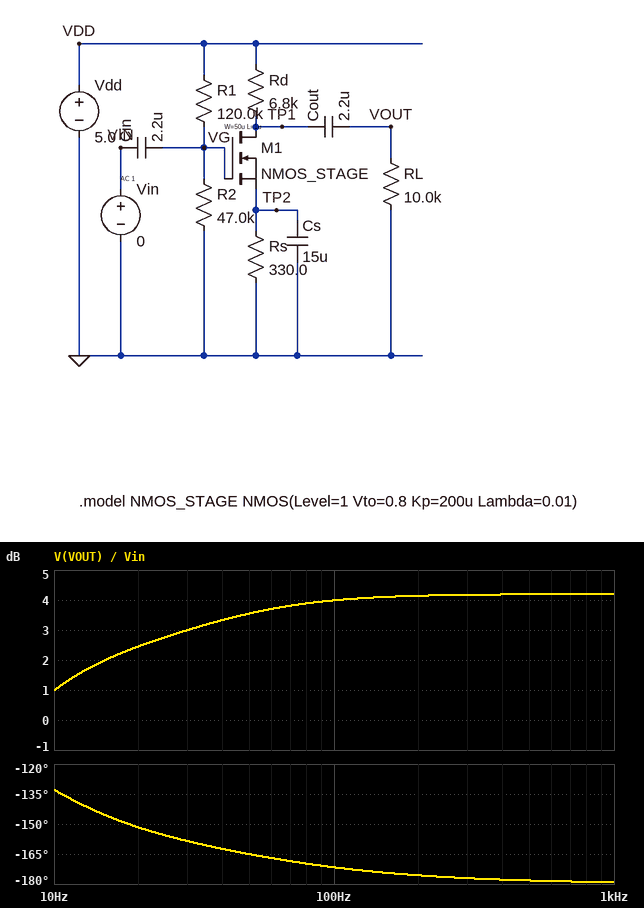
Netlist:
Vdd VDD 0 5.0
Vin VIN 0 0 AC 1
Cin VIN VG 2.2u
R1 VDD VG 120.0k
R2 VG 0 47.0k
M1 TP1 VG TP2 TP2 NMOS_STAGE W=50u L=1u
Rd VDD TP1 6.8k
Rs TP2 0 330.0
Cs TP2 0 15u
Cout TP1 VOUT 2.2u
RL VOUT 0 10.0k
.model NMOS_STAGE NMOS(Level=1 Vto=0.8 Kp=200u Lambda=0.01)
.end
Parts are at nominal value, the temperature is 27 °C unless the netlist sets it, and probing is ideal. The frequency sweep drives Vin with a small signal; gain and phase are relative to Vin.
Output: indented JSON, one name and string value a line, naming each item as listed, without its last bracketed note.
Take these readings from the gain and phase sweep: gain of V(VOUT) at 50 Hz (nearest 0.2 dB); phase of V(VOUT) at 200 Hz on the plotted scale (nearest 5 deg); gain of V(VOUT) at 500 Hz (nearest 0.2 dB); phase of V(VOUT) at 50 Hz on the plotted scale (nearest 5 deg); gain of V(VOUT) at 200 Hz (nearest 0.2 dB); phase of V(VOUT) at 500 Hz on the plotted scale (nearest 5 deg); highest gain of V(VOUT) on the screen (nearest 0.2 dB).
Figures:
{
  "gain of V(VOUT) at 50 Hz": "3.6 dB",
  "phase of V(VOUT) at 200 Hz on the plotted scale": "-175 deg",
  "gain of V(VOUT) at 500 Hz": "4.2 dB",
  "phase of V(VOUT) at 50 Hz on the plotted scale": "-165 deg",
  "gain of V(VOUT) at 200 Hz": "4.2 dB",
  "phase of V(VOUT) at 500 Hz on the plotted scale": "-180 deg",
  "highest gain of V(VOUT) on the screen": "4.2 dB"
}
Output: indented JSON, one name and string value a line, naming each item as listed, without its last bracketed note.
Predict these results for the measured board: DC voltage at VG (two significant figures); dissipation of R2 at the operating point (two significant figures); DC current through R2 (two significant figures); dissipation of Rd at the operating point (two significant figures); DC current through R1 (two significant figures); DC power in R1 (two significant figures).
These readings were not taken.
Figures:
{
  "DC voltage at VG": "1.4 V",
  "dissipation of R2 at the operating point": "42 µW",
  "DC current through R2": "30 µA",
  "dissipation of Rd at the operating point": "3.0 mW",
  "DC current through R1": "30 µA",
  "DC power in R1": "110 µW"
}
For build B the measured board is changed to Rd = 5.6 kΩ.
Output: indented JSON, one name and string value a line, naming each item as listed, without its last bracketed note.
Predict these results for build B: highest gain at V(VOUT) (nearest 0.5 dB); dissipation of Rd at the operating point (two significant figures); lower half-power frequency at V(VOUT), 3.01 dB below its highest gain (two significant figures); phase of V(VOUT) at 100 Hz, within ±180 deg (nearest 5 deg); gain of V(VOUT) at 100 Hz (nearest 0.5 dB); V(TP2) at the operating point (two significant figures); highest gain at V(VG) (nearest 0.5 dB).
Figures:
{
  "highest gain at V(VOUT)": "22.5 dB",
  "dissipation of Rd at the operating point": "2.8 mW",
  "lower half-power frequency at V(VOUT), 3.01 dB below its highest gain": "56 Hz",
  "phase of V(VOUT) at 100 Hz, within ±180 deg": "-160 deg",
  "gain of V(VOUT) at 100 Hz": "21.0 dB",
  "V(TP2) at the operating point": "230 mV",
  "highest gain at V(VG)": "0 dB"
}
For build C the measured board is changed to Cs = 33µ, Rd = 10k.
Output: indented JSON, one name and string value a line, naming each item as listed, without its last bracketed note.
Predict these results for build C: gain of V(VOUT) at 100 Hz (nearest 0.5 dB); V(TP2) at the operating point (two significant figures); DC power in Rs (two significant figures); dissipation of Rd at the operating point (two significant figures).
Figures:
{
  "gain of V(VOUT) at 100 Hz": "-9.5 dB",
  "V(TP2) at the operating point": "160 mV",
  "DC power in Rs": "74 µW",
  "dissipation of Rd at the operating point": "2.2 mW"
}
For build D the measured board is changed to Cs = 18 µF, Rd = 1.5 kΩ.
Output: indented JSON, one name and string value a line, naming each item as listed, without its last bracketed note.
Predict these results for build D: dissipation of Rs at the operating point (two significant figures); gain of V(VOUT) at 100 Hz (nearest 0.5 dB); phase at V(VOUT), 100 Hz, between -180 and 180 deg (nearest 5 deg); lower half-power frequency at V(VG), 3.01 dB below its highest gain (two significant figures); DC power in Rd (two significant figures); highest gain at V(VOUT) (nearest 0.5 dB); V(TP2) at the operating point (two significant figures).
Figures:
{
  "dissipation of Rs at the operating point": "170 µW",
  "gain of V(VOUT) at 100 Hz": "13.0 dB",
  "phase at V(VOUT), 100 Hz, between -180 and 180 deg": "-160 deg",
  "lower half-power frequency at V(VG), 3.01 dB below its highest gain": "2.1 Hz",
  "DC power in Rd": "770 µW",
  "highest gain at V(VOUT)": "14.0 dB",
  "V(TP2) at the operating point": "240 mV"
}
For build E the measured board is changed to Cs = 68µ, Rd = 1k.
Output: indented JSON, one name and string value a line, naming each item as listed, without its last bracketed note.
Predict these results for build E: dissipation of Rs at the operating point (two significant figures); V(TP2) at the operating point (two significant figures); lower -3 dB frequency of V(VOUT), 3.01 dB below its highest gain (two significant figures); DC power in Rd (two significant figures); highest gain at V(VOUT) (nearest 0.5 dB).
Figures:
{
  "dissipation of Rs at the operating point": "170 µW",
  "V(TP2) at the operating point": "240 mV",
  "lower -3 dB frequency of V(VOUT), 3.01 dB below its highest gain": "16 Hz",
  "DC power in Rd": "510 µW",
  "highest gain at V(VOUT)": "11.0 dB"
}
